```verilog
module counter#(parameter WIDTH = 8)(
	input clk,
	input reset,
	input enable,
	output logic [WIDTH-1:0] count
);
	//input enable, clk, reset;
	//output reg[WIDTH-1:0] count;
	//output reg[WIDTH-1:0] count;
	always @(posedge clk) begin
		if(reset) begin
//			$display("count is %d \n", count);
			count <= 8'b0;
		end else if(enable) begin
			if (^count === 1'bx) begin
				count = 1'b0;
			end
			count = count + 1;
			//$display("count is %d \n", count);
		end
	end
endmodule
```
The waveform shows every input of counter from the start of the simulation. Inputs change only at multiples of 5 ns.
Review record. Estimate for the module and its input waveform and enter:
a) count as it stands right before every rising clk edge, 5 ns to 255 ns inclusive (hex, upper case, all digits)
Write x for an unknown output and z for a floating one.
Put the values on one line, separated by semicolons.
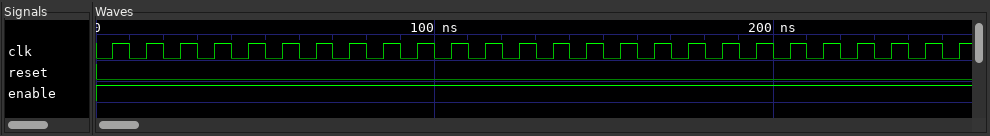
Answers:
x, 01, 02, 03, 04, 05, 06, 07, 08, 09, 0A, 0B, 0C, 0D, 0E, 0F, 10, 11, 12, 13, 14, 15, 16, 17, 18, 19
